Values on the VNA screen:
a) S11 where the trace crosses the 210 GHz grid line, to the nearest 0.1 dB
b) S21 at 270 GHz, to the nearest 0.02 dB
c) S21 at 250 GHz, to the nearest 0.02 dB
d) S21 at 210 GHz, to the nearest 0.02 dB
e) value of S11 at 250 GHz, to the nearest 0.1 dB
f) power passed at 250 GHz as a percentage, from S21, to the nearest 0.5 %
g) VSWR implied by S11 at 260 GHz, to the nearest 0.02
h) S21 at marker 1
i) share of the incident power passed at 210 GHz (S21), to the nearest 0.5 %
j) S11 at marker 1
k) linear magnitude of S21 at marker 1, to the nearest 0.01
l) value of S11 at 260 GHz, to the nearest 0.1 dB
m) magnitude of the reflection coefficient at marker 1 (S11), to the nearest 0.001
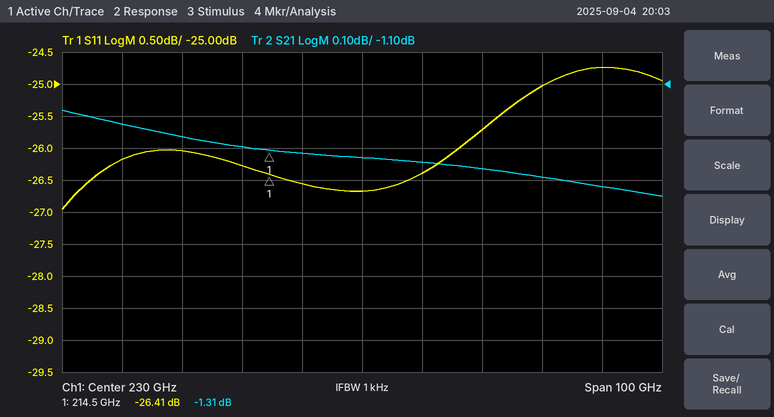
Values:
-26.3 dB
-1.42 dB
-1.36 dB
-1.30 dB
-25.7 dB
73.0 %
1.12
-1.31 dB
74.0 %
-26.41 dB
0.86
-25.0 dB
0.048
